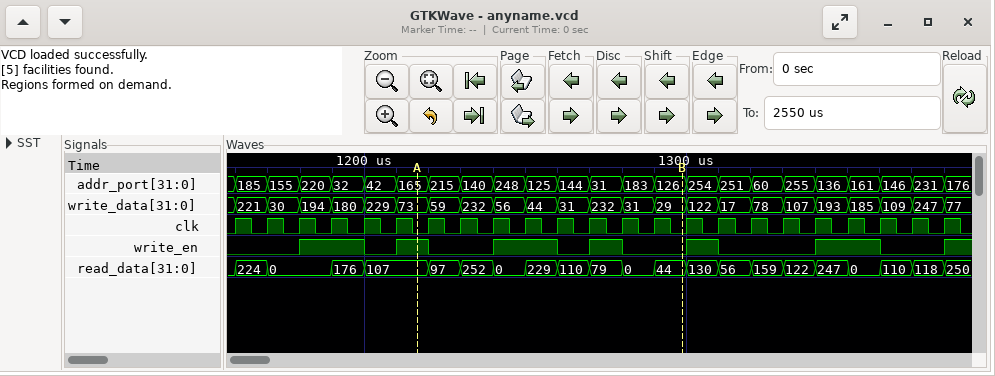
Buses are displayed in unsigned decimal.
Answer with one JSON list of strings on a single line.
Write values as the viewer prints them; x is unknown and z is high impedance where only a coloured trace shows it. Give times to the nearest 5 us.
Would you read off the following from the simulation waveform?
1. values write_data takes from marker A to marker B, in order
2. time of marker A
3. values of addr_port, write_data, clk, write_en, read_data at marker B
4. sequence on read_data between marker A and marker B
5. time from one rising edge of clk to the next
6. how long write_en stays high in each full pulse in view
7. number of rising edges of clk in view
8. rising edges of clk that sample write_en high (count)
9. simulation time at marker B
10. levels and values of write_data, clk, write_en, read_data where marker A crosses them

["73, 59, 232, 56, 44, 31, 232, 31, 29", "1215 us", "addr_port=126, write_data=29, clk=0, write_en=0, read_data=44", "107, 97, 252, 0, 229, 110, 79, 0, 44", "10 us", "20 us, 10 us, 20 us, 10 us, 10 us, 20 us", "23", "9", "1300 us", "write_data=73, clk=0, write_en=1, read_data=107"]
